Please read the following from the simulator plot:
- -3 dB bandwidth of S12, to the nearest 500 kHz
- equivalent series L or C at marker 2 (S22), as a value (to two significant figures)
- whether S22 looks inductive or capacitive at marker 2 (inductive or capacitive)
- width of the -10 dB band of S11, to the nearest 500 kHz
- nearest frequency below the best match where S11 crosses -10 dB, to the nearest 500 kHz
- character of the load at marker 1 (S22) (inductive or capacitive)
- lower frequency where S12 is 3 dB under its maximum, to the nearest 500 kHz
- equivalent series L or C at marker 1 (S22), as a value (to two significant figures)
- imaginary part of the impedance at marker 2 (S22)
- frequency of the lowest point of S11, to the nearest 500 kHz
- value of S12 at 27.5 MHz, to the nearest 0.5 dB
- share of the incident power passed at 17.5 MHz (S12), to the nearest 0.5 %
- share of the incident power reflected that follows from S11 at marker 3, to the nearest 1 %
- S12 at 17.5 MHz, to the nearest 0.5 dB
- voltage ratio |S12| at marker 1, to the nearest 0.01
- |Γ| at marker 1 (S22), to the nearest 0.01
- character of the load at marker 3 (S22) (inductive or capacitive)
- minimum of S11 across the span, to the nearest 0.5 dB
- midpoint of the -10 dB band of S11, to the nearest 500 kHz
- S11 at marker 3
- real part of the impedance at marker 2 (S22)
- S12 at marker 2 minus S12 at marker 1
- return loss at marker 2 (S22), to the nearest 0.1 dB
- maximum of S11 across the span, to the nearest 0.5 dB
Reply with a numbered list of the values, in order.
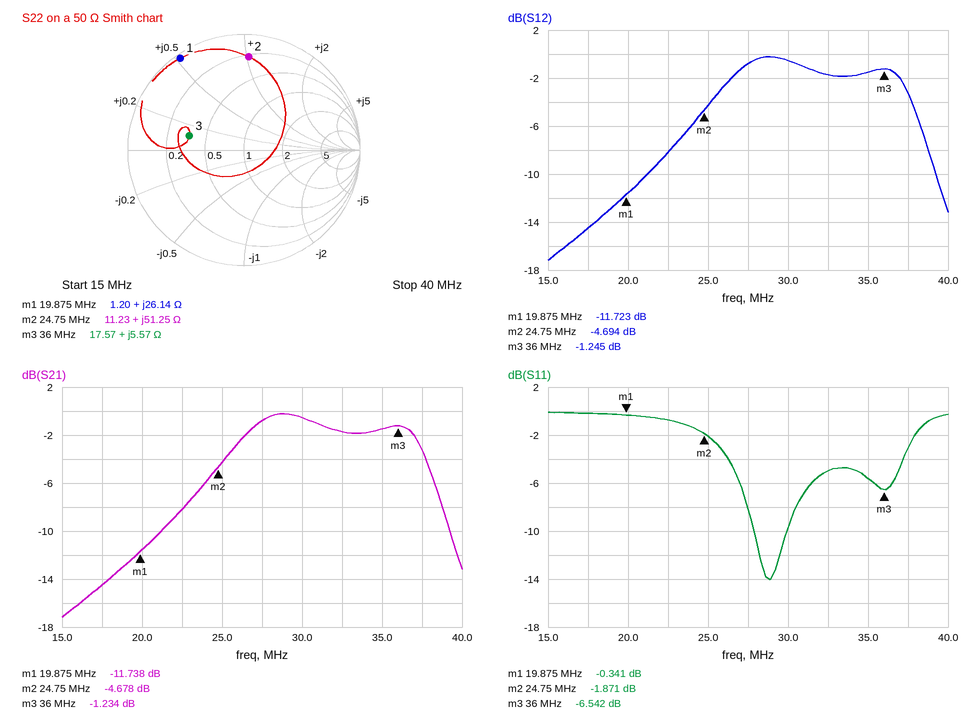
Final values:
1. 12.0 MHz
2. 330 nH
3. inductive
4. 2.0 MHz
5. 28.0 MHz
6. inductive
7. 25.5 MHz
8. 210 nH
9. +51.25 Ω
10. 29.0 MHz
11. -1.0 dB
12. 3.5 %
13. 22 %
14. -14.5 dB
15. 0.26
16. 0.96
17. inductive
18. -14.0 dB
19. 29.0 MHz
20. -6.542 dB
21. 11.23 Ω
22. 7.029 dB
23. 1.9 dB
24. 0.0 dB
